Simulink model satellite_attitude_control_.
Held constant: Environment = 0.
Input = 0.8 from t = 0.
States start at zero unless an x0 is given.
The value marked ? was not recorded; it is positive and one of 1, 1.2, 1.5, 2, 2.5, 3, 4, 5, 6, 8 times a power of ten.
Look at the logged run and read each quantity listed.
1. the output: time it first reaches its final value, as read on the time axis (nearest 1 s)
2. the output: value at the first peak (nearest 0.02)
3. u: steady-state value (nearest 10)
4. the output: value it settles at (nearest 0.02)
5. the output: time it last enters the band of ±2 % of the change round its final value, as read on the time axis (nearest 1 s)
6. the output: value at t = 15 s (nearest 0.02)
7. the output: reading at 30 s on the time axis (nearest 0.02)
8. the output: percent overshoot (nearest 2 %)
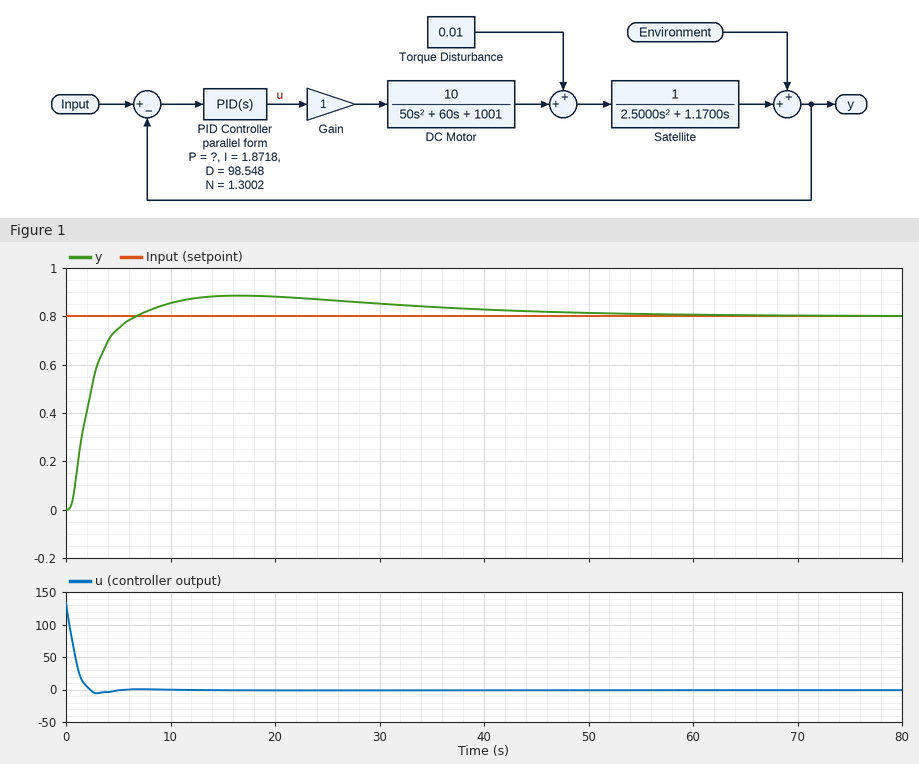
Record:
7 s
0.88
0
0.80
48 s
0.88
0.86
10 %
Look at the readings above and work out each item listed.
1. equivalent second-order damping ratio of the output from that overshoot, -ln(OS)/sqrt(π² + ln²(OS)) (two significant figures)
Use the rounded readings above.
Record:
0.59
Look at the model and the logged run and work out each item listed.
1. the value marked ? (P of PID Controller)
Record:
40
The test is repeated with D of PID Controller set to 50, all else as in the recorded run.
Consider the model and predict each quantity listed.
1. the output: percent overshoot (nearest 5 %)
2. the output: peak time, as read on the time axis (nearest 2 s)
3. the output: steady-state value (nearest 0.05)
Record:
15 %
12 s
0.80
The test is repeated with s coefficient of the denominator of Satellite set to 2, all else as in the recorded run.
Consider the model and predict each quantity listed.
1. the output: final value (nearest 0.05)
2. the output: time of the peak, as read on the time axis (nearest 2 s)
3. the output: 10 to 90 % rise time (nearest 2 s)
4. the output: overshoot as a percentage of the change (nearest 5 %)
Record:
0.80
24 s
8 s
15 %
